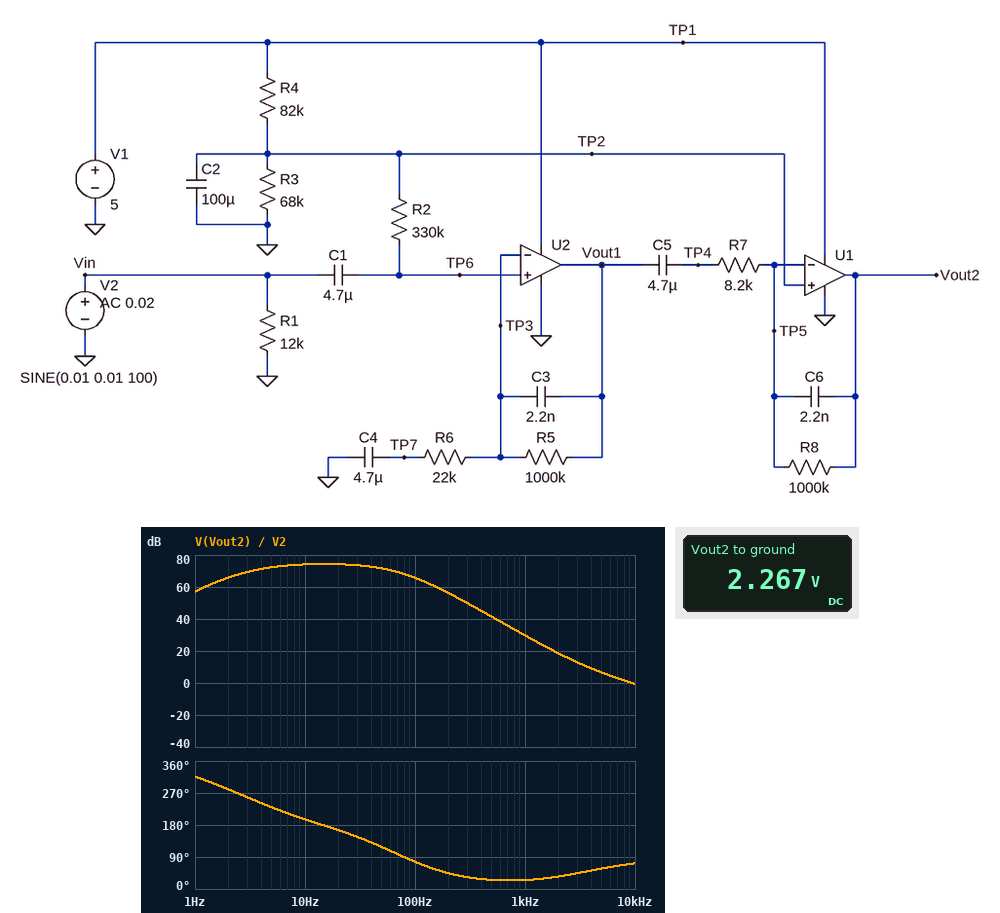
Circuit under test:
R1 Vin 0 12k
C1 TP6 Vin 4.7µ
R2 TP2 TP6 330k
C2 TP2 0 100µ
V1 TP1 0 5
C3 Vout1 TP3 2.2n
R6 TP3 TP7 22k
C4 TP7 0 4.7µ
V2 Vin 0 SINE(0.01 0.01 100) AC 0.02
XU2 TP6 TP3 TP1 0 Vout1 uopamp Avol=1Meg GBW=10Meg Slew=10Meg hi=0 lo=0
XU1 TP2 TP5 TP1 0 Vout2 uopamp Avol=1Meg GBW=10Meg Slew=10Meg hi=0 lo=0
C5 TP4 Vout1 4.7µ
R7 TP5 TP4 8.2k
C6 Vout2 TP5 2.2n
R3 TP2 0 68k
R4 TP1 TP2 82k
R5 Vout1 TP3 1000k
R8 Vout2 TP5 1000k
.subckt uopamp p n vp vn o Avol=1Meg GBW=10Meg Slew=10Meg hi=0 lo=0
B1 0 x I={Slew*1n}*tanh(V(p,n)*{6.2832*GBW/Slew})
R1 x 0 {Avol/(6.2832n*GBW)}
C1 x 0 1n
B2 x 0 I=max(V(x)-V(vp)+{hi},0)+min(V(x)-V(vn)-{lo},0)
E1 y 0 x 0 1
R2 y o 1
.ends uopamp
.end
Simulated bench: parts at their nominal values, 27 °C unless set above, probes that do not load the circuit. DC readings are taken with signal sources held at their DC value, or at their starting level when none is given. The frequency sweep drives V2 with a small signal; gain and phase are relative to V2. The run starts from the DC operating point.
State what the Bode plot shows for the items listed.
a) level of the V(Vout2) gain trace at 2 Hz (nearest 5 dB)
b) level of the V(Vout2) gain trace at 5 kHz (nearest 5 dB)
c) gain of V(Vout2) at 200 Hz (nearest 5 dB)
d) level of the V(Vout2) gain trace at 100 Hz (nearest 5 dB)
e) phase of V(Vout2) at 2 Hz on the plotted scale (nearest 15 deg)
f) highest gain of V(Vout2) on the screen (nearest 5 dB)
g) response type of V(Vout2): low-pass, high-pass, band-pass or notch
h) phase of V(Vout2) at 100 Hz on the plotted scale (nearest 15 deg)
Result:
65 dB
5 dB
55 dB
65 dB
285 deg
75 dB
band-pass
75 deg
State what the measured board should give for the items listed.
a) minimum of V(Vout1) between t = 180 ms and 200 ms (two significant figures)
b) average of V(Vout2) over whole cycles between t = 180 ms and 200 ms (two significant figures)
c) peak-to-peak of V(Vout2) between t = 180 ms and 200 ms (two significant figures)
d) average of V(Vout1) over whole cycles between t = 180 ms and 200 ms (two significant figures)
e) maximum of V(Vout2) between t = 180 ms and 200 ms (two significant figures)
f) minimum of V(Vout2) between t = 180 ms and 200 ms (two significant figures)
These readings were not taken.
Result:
2.0 V
2.5 V
5.0 V
2.3 V
5.0 V
-9.2 mV
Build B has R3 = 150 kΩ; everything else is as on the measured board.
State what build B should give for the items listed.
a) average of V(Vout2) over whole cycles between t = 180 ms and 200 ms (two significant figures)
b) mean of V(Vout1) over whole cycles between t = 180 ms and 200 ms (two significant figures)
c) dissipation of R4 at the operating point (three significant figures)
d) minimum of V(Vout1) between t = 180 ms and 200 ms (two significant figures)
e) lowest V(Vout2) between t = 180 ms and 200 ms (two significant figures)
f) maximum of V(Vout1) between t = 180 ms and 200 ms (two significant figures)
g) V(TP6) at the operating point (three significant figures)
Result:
2.7 V
3.2 V
38.1 µW
3.0 V
-8.8 mV
3.5 V
3.23 V
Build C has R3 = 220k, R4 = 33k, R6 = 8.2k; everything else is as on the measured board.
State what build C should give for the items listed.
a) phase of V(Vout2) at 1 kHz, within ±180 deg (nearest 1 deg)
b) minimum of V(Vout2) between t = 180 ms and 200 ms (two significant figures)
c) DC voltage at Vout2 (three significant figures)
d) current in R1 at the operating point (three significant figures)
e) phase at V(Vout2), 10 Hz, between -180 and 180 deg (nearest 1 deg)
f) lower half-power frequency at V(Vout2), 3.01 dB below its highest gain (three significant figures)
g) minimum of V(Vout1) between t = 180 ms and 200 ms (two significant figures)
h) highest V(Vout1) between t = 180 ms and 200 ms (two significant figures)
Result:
15 deg
-10 mV
4.35 V
833 nA
-150 deg
5.46 Hz
3.6 V
5.0 V
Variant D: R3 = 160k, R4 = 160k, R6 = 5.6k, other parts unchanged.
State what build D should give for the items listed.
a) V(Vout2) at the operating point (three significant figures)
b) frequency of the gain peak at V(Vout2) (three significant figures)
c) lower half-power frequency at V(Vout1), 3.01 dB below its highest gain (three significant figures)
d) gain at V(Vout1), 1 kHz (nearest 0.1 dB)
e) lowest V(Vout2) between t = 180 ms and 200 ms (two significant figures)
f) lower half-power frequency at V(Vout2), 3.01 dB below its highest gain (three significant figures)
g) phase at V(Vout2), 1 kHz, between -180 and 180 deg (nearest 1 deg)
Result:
2.50 V
19.3 Hz
5.23 Hz
22.3 dB
-10 mV
6.54 Hz
13 deg
